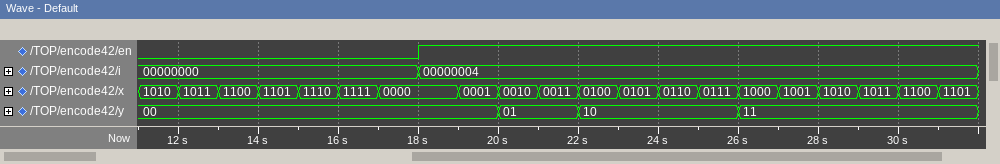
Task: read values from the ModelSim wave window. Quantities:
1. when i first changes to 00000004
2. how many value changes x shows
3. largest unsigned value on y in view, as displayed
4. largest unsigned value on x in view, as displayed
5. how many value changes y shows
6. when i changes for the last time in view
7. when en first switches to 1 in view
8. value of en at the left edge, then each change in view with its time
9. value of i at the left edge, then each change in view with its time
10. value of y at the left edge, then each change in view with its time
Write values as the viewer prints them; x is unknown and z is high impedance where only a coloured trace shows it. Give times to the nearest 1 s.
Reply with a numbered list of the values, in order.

1. 18 s
2. 19
3. 11
4. 1111
5. 3
6. 18 s
7. 18 s
8. 0, 1 at 18 s
9. 00000000, 00000004 at 18 s
10. 00, 01 at 20 s, 10 at 22 s, 11 at 26 s
